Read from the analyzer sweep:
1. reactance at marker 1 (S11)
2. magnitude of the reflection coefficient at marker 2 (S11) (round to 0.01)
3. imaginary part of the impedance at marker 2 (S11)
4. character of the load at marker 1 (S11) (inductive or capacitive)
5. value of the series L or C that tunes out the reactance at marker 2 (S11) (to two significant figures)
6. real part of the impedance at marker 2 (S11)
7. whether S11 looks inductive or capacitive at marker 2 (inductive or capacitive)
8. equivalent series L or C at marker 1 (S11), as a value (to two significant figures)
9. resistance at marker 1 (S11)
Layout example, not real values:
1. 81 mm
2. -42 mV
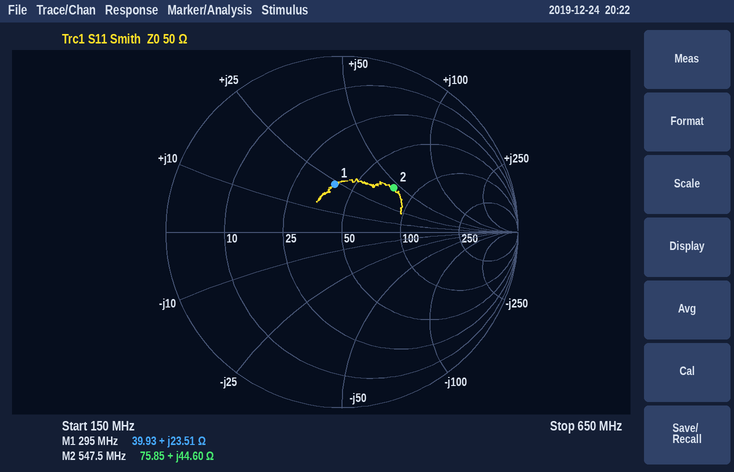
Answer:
1. +23.51 Ω
2. 0.39
3. +44.60 Ω
4. inductive
5. 6.5 pF
6. 75.85 Ω
7. inductive
8. 13 nH
9. 39.93 Ω
